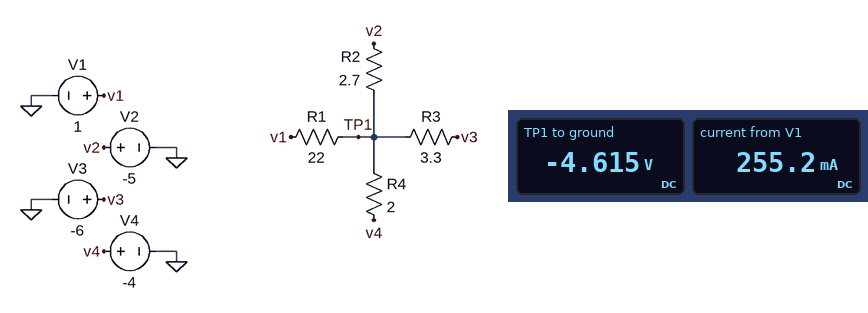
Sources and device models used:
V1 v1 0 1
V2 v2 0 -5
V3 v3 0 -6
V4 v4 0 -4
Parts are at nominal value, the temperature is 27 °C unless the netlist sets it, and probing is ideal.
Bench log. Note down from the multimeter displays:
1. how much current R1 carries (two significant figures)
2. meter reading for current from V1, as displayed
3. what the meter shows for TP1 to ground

260 mA
255.2 mA
-4.615 V
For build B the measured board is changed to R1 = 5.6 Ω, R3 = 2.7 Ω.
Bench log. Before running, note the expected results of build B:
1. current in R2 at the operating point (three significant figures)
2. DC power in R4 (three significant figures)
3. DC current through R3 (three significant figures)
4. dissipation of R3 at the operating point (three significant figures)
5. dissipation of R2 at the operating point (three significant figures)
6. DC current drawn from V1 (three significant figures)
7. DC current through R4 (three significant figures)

313 mA
11.8 mW
684 mA
1.26 W
265 mW
920 mA
76.9 mA
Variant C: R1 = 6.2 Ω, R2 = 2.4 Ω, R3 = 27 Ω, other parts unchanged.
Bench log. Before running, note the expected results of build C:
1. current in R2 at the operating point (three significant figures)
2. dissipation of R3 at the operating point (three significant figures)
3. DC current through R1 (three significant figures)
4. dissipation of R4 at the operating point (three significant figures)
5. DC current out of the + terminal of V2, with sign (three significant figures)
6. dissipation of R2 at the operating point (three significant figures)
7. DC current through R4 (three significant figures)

535 mA
193 mW
761 mA
40.1 mW
-535 mA
686 mW
142 mA
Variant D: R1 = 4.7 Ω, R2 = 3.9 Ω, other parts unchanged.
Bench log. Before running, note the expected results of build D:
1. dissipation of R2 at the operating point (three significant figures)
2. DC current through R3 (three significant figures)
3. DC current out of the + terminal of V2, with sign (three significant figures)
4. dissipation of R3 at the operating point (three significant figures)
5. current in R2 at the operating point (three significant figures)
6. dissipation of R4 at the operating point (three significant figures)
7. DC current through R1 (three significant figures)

344 mW
654 mA
-297 mA
1.41 W
297 mA
12.5 mW
1.03 A
